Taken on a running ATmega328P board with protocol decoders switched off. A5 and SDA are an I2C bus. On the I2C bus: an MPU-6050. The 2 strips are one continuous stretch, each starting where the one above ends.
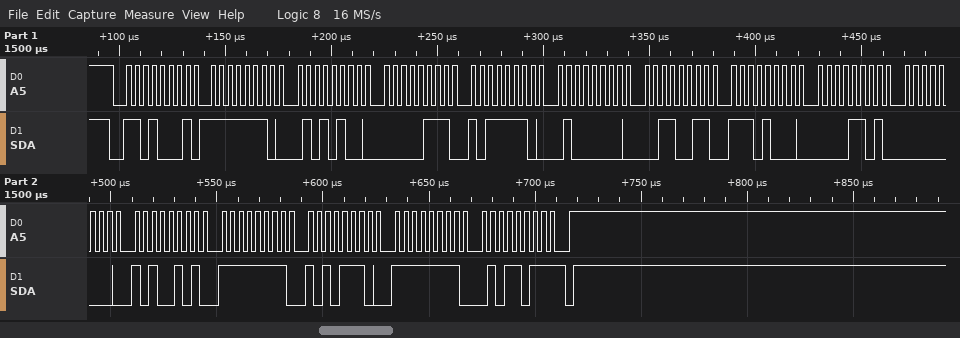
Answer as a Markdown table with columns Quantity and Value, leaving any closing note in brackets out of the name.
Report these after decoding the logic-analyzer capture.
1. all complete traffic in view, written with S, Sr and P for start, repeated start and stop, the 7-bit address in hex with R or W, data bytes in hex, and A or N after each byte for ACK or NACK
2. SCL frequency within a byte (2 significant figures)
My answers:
| Quantity | Value |
|---|---|
| all complete traffic in view, written with S, Sr and P for start, repeated start and stop, the 7-bit address in hex with R or W, data bytes in hex, and A or N after each byte for ACK or NACK | S 68R A FE A 54 A 07 A BE A 40 A 33 A E8 A 0D A 00 A A5 A FF A AE A FF A 5B N P |
| SCL frequency within a byte | 250 kHz |
